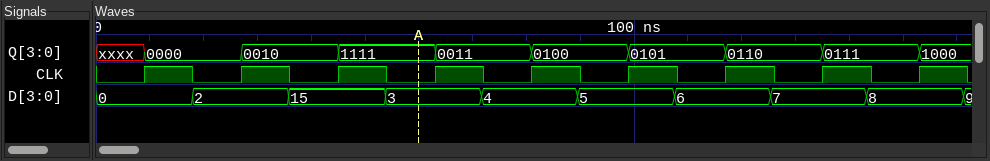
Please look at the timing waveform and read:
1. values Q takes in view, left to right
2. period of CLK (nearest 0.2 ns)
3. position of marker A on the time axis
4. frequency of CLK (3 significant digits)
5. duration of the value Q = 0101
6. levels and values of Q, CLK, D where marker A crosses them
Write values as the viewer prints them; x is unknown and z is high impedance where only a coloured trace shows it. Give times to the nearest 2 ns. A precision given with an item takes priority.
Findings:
xxxx, 0000, 0010, 1111, 0011, 0100, 0101, 0110, 0111, 1000
18 ns
60 ns
55.6 MHz
18 ns
Q=1111, CLK=0, D=3
